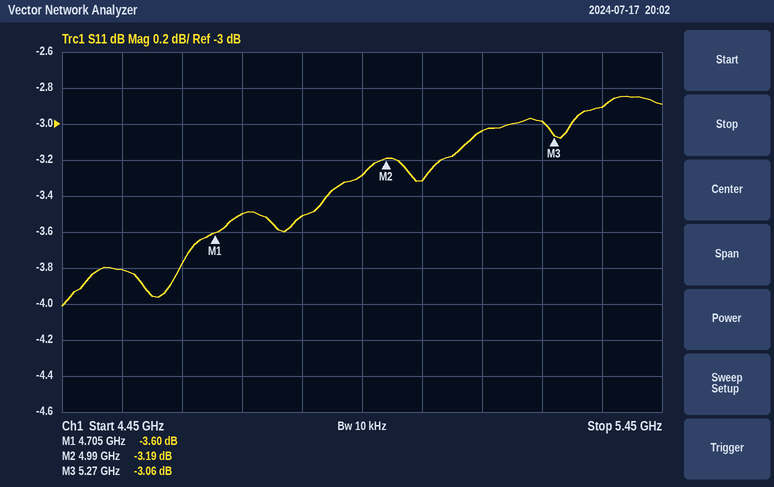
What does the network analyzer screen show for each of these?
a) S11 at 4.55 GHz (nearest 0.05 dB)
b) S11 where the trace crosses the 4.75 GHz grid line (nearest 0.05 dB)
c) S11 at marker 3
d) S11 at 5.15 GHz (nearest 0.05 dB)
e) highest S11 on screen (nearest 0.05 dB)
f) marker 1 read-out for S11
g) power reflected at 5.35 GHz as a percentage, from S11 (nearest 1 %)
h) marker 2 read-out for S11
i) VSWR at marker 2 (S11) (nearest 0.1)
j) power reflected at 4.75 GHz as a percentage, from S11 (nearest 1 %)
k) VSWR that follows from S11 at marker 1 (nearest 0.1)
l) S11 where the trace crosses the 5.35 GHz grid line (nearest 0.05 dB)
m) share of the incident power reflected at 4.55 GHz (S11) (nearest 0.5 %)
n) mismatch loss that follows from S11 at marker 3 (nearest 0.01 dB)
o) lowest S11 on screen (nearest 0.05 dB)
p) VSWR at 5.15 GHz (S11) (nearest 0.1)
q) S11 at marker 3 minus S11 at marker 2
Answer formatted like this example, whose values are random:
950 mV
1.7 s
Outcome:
-3.80 dB
-3.50 dB
-3.06 dB
-3.05 dB
-2.85 dB
-3.60 dB
51 %
-3.19 dB
5.5
45 %
4.9
-2.90 dB
41.5 %
2.96 dB
-4.00 dB
5.8
0.13 dB
